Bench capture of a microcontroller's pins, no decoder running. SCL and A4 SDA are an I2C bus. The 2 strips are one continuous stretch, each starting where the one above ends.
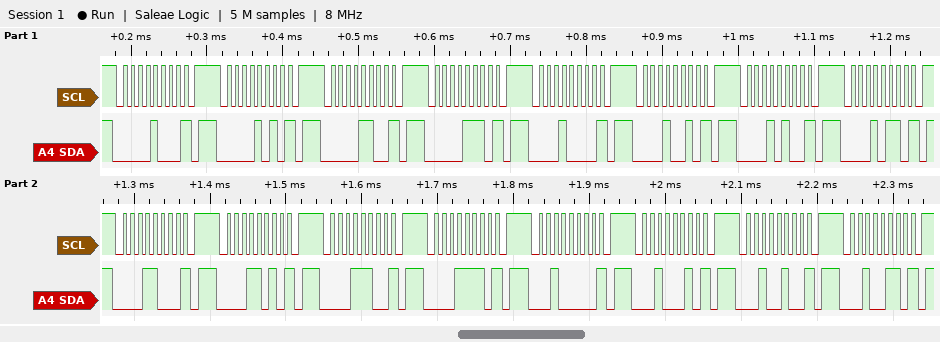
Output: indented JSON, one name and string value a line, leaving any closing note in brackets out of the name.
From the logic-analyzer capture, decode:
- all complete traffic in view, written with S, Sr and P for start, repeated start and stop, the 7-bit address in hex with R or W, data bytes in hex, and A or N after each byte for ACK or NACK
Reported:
{
  "all complete traffic in view, written with S, Sr and P for start, repeated start and stop, the 7-bit address in hex with R or W, data bytes in hex, and A or N after each byte for ACK or NACK": "S 04W N P S 05W N P S 06W N P S 07W N P S 08W N P S 09W N P S 0AW N P S 0BW N P S 0CW N P S 0DW N P S 0EW N P S 0FW N P S 10W N P S 11W N P S 12W N P S 13W N P"
}
